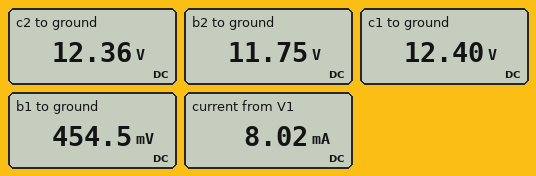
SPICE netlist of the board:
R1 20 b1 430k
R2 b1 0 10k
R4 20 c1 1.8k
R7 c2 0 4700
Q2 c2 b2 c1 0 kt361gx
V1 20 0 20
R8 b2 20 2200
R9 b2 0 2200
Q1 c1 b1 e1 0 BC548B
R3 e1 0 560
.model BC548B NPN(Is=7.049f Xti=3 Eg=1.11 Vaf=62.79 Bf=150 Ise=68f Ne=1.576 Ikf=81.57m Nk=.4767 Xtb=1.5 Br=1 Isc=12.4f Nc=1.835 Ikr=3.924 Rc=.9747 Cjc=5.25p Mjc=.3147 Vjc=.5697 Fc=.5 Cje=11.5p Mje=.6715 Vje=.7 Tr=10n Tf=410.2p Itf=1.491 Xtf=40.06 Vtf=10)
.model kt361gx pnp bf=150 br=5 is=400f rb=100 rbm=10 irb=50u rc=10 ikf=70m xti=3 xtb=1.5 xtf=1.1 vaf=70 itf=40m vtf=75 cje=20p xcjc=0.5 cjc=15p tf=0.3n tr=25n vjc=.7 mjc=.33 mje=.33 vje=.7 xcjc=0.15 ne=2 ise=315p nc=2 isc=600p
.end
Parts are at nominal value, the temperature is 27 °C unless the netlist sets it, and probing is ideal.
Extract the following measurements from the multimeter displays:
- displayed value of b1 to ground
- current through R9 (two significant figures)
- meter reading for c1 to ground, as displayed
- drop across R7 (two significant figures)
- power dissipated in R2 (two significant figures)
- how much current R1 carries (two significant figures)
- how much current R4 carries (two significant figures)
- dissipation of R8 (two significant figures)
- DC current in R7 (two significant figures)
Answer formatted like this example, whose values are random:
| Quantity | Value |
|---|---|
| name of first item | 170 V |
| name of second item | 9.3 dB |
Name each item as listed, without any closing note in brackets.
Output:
| Quantity | Value |
|---|---|
| displayed value of b1 to ground | 454.5 mV |
| current through R9 | 5.3 mA |
| meter reading for c1 to ground, as displayed | 12.40 V |
| drop across R7 | 12 V |
| power dissipated in R2 | 21 µW |
| how much current R1 carries | 45 µA |
| how much current R4 carries | 4.2 mA |
| dissipation of R8 | 31 mW |
| DC current in R7 | 2.6 mA |
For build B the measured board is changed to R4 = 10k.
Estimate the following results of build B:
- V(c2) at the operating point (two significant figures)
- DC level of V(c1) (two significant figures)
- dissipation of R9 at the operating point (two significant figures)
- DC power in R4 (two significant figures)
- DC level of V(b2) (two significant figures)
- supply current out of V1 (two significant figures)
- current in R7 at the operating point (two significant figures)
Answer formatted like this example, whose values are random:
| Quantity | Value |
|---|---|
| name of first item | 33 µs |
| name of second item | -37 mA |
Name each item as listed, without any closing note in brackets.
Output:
| Quantity | Value |
|---|---|
| V(c2) at the operating point | 4.3 V |
| DC level of V(c1) | 11 V |
| dissipation of R9 at the operating point | 46 mW |
| DC power in R4 | 8.9 mW |
| DC level of V(b2) | 10 V |
| supply current out of V1 | 5.5 mA |
| current in R7 at the operating point | 920 µA |
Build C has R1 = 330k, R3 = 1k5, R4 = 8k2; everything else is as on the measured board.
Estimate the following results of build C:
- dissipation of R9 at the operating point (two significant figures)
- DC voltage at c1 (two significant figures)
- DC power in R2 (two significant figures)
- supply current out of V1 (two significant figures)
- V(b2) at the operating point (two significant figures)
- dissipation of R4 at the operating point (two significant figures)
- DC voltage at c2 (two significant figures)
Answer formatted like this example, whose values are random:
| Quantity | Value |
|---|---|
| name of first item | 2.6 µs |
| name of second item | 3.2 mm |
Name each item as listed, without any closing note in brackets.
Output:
| Quantity | Value |
|---|---|
| dissipation of R9 at the operating point | 46 mW |
| DC voltage at c1 | 11 V |
| DC power in R2 | 34 µW |
| supply current out of V1 | 5.7 mA |
| V(b2) at the operating point | 10 V |
| dissipation of R4 at the operating point | 11 mW |
| DC voltage at c2 | 5.2 V |
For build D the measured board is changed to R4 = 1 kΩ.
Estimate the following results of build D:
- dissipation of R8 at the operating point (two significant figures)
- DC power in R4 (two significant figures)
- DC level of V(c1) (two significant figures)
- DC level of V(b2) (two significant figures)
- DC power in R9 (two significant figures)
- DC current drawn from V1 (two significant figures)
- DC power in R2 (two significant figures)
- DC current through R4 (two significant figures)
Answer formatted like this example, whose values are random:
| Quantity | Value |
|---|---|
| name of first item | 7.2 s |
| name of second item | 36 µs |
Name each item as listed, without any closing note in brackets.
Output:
| Quantity | Value |
|---|---|
| dissipation of R8 at the operating point | 20 mW |
| DC power in R4 | 36 mW |
| DC level of V(c1) | 14 V |
| DC level of V(b2) | 13 V |
| DC power in R9 | 81 mW |
| DC current drawn from V1 | 9.1 mA |
| DC power in R2 | 21 µW |
| DC current through R4 | 6.0 mA |
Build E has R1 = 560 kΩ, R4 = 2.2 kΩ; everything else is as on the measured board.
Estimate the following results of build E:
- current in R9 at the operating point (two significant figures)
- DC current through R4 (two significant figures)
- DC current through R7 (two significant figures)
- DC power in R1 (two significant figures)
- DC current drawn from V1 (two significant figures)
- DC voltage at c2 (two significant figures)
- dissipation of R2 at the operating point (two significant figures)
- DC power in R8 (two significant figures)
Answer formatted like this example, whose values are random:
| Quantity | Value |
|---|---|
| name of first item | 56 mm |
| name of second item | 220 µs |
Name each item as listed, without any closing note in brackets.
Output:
| Quantity | Value |
|---|---|
| current in R9 at the operating point | 5.1 mA |
| DC current through R4 | 3.7 mA |
| DC current through R7 | 2.5 mA |
| DC power in R1 | 690 µW |
| DC current drawn from V1 | 7.7 mA |
| DC voltage at c2 | 12 V |
| dissipation of R2 at the operating point | 12 µW |
| DC power in R8 | 35 mW |
